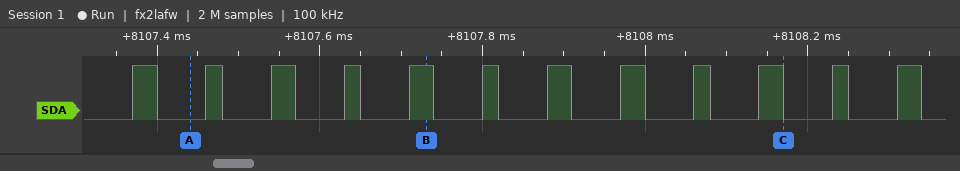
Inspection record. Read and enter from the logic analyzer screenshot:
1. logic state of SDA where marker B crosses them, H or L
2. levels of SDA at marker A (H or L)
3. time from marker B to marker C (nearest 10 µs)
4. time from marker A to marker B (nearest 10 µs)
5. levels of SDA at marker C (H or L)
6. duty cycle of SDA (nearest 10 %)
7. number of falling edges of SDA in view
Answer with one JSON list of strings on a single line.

["SDA=H", "SDA=L", "440 µs", "290 µs", "SDA=L", "30 %", "12"]
